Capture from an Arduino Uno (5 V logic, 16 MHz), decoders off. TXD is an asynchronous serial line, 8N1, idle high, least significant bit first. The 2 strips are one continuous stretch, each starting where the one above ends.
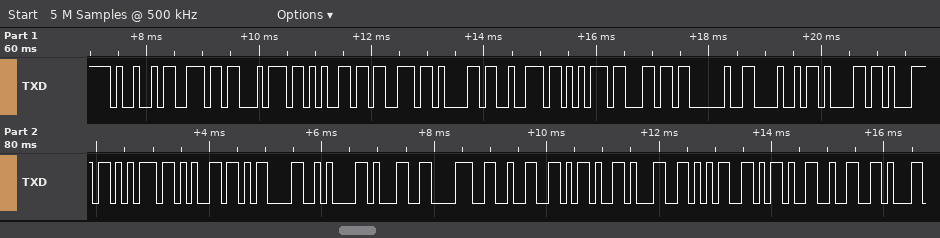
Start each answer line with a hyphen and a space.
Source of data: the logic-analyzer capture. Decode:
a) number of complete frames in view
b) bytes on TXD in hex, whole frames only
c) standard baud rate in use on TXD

- 25
- 0x49 0x6E 0x74 0x65 0x73 0x61 0x72 0x75 0x6C 0x20 0x48 0x61 0x71 0x75 0x65 0x0D 0x0A 0x31 0x38 0x32 0x2D 0x31 0x35 0x2D 0x32
- 9600 baud
